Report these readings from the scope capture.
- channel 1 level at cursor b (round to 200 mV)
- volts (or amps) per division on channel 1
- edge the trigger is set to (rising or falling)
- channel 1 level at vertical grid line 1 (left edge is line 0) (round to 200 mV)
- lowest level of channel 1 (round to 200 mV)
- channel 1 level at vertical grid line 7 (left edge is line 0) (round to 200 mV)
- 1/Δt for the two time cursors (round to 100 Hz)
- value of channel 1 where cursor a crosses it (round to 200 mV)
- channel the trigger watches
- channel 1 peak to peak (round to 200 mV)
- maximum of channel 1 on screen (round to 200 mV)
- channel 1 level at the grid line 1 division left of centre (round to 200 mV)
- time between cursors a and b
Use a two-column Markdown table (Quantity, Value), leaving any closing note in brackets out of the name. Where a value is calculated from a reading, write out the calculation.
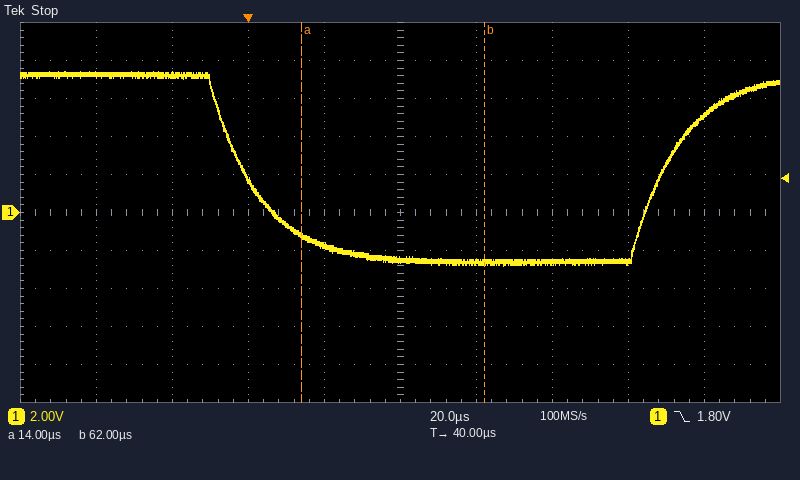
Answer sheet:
| Quantity | Value |
|---|---|
| channel 1 level at cursor b | -2.6 V |
| volts (or amps) per division on channel 1 | 2 V |
| edge the trigger is set to | falling |
| channel 1 level at vertical grid line 1 (left edge is line 0) | 7.2 V |
| lowest level of channel 1 | -2.8 V |
| channel 1 level at vertical grid line 7 (left edge is line 0) | -2.6 V |
| 1/Δt for the two time cursors | 1 / 48 µs ≈ 20.8 kHz |
| value of channel 1 where cursor a crosses it | -1.2 V |
| channel the trigger watches | channel 1 |
| channel 1 peak to peak | 7.4 V − (-2.8 V) = 10.2 V |
| maximum of channel 1 on screen | 7.4 V |
| channel 1 level at the grid line 1 division left of centre | -1.8 V |
| time between cursors a and b | 62 µs − (14 µs) = 48 µs |
